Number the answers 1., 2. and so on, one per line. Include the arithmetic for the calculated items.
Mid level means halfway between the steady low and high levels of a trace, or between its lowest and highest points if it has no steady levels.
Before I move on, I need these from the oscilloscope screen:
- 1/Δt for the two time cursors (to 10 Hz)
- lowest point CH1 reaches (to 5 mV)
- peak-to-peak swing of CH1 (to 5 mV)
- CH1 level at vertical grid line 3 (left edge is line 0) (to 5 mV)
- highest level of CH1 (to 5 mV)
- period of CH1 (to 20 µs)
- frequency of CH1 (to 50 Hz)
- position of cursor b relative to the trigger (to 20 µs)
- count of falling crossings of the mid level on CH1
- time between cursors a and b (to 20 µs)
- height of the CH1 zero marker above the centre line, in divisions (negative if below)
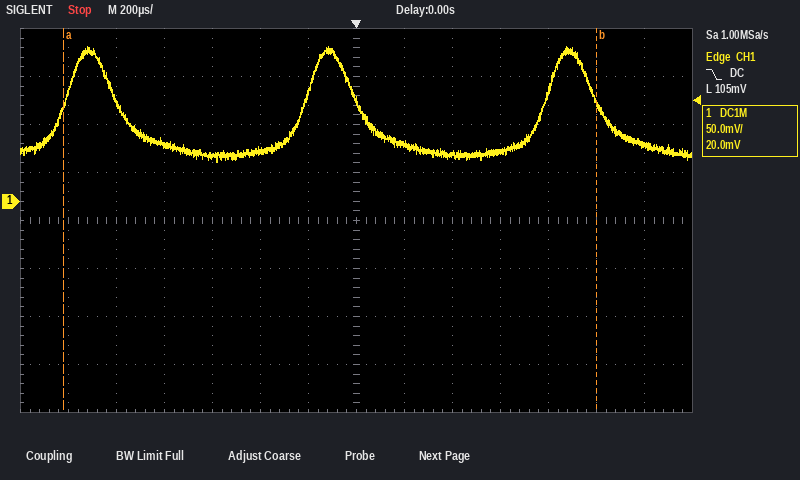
1. 1 / 2.22 ms ≈ 450 Hz
2. 40 mV
3. 160 mV − (40 mV) = 120 mV
4. 60 mV
5. 160 mV
6. 1.00 ms
7. 1 / 1.00 ms ≈ 1.00 kHz
8. +1.00 ms
9. 3
10. 2.22 ms
11. +0.4 div
